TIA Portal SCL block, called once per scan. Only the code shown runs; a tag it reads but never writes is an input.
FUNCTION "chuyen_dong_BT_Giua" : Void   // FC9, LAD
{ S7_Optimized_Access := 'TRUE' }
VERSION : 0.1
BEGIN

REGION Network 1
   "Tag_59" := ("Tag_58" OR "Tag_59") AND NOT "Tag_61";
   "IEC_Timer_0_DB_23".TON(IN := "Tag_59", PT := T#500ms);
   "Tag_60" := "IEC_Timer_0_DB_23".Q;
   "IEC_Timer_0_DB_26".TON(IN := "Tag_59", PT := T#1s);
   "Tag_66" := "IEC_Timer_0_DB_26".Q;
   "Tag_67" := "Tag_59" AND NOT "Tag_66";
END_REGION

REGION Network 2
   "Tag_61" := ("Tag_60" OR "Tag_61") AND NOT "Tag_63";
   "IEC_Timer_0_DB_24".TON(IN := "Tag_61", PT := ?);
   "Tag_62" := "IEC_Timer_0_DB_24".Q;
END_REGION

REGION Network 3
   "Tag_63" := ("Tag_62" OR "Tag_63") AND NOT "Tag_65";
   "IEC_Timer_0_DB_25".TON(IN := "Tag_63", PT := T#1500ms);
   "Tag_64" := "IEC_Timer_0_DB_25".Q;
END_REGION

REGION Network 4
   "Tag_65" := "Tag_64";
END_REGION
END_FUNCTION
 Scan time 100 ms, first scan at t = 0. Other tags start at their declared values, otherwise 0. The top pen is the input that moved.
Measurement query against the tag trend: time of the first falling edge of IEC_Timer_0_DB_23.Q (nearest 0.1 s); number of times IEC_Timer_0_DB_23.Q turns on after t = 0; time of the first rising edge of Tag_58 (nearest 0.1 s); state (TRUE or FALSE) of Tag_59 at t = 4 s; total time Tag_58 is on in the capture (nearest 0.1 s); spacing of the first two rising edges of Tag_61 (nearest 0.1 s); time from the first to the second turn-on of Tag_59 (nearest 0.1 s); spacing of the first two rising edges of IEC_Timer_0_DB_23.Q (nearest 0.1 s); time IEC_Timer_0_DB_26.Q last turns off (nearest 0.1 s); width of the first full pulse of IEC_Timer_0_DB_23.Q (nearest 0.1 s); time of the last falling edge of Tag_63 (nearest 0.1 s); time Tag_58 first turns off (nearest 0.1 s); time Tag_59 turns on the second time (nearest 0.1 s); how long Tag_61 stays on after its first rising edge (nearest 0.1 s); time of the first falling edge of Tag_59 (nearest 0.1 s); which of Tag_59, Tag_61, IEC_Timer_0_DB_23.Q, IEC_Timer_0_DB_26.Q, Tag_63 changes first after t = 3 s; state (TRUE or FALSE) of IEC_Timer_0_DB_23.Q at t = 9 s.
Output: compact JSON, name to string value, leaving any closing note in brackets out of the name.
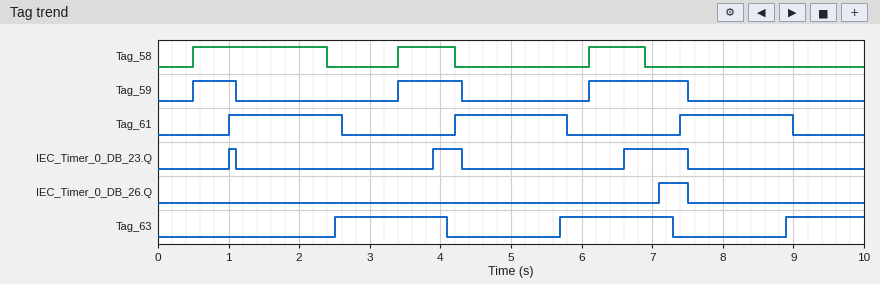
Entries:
{"time of the first falling edge of IEC_Timer_0_DB_23.Q": "1.1 s", "number of times IEC_Timer_0_DB_23.Q turns on after t = 0": "3", "time of the first rising edge of Tag_58": "0.5 s", "state (TRUE or FALSE) of Tag_59 at t = 4 s": "TRUE", "total time Tag_58 is on in the capture": "3.5 s", "spacing of the first two rising edges of Tag_61": "3.2 s", "time from the first to the second turn-on of Tag_59": "2.9 s", "spacing of the first two rising edges of IEC_Timer_0_DB_23.Q": "2.9 s", "time IEC_Timer_0_DB_26.Q last turns off": "7.5 s", "width of the first full pulse of IEC_Timer_0_DB_23.Q": "0.1 s", "time of the last falling edge of Tag_63": "7.3 s", "time Tag_58 first turns off": "2.4 s", "time Tag_59 turns on the second time": "3.4 s", "how long Tag_61 stays on after its first rising edge": "1.6 s", "time of the first falling edge of Tag_59": "1.1 s", "which of Tag_59, Tag_61, IEC_Timer_0_DB_23.Q, IEC_Timer_0_DB_26.Q, Tag_63 changes first after t = 3 s": "Tag_59", "state (TRUE or FALSE) of IEC_Timer_0_DB_23.Q at t = 9 s": "FALSE"}
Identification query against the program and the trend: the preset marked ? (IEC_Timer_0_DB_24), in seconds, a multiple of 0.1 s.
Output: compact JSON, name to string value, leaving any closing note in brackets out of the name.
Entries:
{"the preset marked ? (IEC_Timer_0_DB_24), in seconds, a multiple of 0.1 s": "1.5 s"}
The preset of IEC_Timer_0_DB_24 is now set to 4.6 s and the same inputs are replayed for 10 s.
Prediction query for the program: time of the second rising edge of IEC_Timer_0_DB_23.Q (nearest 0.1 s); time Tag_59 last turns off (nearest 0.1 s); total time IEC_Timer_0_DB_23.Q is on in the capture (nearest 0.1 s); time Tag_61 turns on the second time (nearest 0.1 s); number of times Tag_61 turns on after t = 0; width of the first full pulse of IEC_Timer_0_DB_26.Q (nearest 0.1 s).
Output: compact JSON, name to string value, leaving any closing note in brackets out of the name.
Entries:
{"time of the second rising edge of IEC_Timer_0_DB_23.Q": "6.6 s", "time Tag_59 last turns off": "7.4 s", "total time IEC_Timer_0_DB_23.Q is on in the capture": "0.9 s", "time Tag_61 turns on the second time": "7.3 s", "number of times Tag_61 turns on after t = 0": "2", "width of the first full pulse of IEC_Timer_0_DB_26.Q": "0.3 s"}
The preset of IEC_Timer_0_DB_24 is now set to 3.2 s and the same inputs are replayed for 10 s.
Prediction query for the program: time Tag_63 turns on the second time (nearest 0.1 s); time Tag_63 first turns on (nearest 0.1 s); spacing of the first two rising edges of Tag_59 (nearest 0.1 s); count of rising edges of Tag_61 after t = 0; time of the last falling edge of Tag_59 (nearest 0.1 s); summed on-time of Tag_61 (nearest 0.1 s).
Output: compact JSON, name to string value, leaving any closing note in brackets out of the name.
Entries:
{"time Tag_63 turns on the second time": "9.8 s", "time Tag_63 first turns on": "4.2 s", "spacing of the first two rising edges of Tag_59": "5.6 s", "count of rising edges of Tag_61 after t = 0": "2", "time of the last falling edge of Tag_59": "6.7 s", "summed on-time of Tag_61": "6.6 s"}
